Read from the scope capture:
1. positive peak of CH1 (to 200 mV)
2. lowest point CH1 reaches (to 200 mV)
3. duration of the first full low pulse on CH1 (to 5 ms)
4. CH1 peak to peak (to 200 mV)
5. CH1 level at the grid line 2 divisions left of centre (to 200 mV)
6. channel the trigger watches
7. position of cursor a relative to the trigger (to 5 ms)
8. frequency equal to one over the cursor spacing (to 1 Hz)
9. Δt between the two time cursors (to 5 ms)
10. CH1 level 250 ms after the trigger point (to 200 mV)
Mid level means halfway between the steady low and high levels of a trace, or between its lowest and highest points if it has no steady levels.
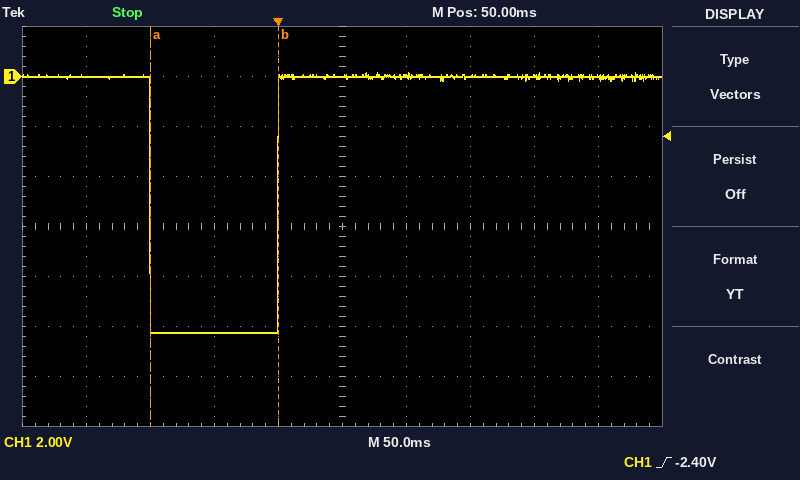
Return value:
200 mV
-10.2 V
100 ms
10.4 V
-10.2 V
CH1
-100 ms
10 Hz
100 ms
0.0 V
